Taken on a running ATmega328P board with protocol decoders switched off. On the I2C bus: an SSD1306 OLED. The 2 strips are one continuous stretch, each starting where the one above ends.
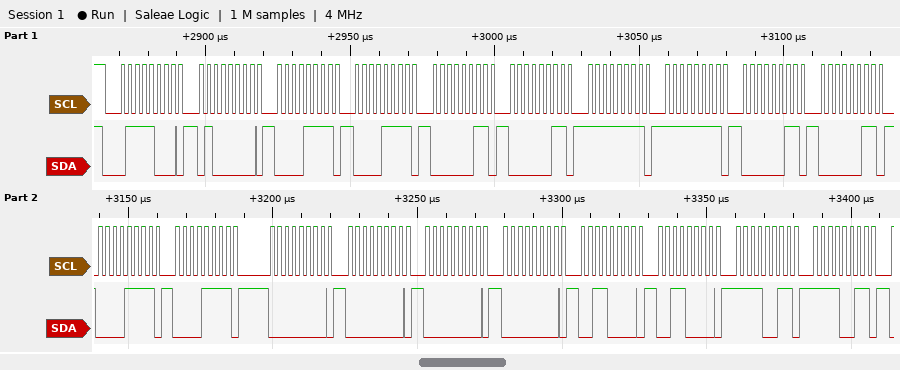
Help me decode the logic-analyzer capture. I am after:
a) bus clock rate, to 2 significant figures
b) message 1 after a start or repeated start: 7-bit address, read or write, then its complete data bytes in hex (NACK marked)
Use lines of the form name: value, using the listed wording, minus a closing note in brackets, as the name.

bus clock rate, to 2 significant figures: 400 kHz
message 1 after a start or repeated start: 7-bit address, read or write, then its complete data bytes in hex: 0x3C write: 40 0F 0F 03 03 FF FF 03 03 0F 0F 00 00 00 00 30 30 F3 F3
